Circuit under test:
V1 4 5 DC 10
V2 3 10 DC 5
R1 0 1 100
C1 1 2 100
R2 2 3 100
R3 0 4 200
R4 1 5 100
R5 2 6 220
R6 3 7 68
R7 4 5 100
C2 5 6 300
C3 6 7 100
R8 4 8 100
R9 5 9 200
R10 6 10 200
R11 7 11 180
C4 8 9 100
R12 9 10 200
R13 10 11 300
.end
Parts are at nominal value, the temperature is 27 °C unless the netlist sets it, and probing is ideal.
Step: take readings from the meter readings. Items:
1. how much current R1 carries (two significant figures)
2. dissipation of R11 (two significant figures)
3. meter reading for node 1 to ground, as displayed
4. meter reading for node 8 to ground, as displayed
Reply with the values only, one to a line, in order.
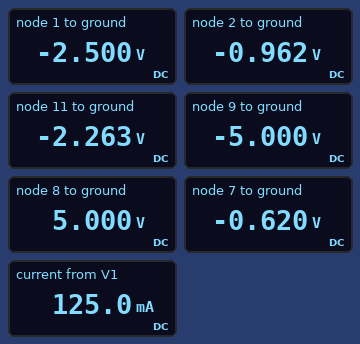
25 mA
15 mW
-2.500 V
5.000 V
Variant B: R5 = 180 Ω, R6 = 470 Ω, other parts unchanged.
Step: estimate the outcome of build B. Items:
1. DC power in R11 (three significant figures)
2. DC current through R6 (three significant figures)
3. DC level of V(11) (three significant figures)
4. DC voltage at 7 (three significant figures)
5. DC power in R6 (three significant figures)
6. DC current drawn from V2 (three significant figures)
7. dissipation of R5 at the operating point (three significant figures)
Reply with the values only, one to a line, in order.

4.99 mW
5.26 mA
-3.42 V
-2.47 V
13.0 mW
15.7 mA
19.5 mW
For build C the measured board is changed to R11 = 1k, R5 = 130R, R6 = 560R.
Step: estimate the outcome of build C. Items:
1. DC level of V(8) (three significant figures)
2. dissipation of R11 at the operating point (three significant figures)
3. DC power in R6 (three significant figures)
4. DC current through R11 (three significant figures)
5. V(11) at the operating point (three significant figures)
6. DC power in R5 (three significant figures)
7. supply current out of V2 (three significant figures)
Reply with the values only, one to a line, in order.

5.00 V
7.23 mW
4.05 mW
2.69 mA
-4.19 V
17.6 mW
14.3 mA
